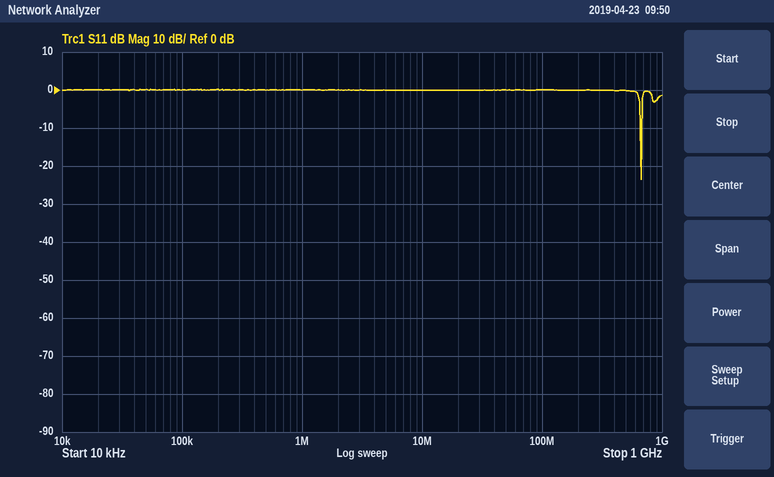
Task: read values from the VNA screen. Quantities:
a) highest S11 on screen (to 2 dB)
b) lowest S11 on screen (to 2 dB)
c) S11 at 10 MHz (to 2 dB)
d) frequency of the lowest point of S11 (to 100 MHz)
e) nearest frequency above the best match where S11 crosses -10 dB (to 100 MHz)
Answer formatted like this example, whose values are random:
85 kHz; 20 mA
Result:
0 dB; -24 dB; 0 dB; 700 MHz; 700 MHz
